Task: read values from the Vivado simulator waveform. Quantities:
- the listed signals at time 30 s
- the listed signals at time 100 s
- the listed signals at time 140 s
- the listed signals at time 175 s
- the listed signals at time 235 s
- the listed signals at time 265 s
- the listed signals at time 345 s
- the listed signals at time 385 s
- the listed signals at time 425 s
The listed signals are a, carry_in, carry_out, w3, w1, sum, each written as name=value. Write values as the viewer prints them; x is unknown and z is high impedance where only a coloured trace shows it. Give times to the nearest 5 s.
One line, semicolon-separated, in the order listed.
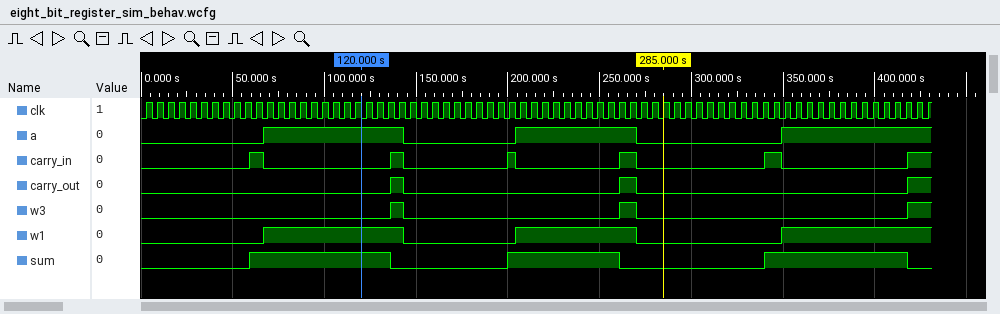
a=0, carry_in=0, carry_out=0, w3=0, w1=0, sum=0; a=1, carry_in=0, carry_out=0, w3=0, w1=1, sum=1; a=1, carry_in=1, carry_out=1, w3=1, w1=1, sum=0; a=0, carry_in=0, carry_out=0, w3=0, w1=0, sum=0; a=1, carry_in=0, carry_out=0, w3=0, w1=1, sum=1; a=1, carry_in=1, carry_out=1, w3=1, w1=1, sum=0; a=0, carry_in=1, carry_out=0, w3=0, w1=0, sum=1; a=1, carry_in=0, carry_out=0, w3=0, w1=1, sum=1; a=1, carry_in=1, carry_out=1, w3=1, w1=1, sum=0
